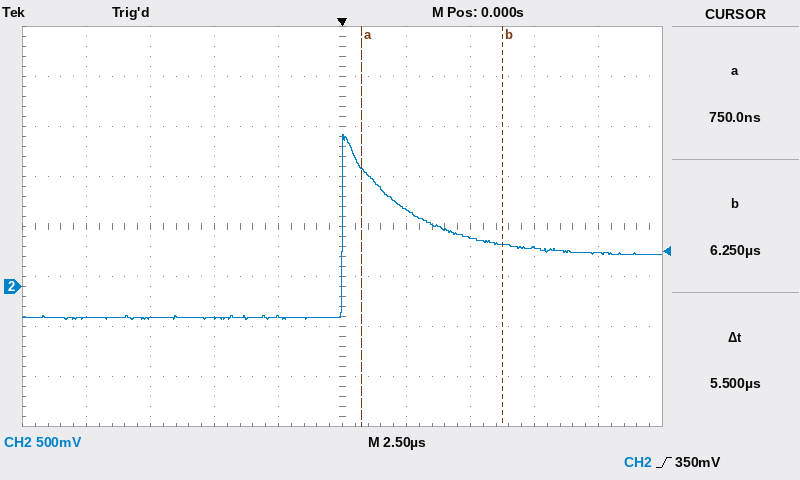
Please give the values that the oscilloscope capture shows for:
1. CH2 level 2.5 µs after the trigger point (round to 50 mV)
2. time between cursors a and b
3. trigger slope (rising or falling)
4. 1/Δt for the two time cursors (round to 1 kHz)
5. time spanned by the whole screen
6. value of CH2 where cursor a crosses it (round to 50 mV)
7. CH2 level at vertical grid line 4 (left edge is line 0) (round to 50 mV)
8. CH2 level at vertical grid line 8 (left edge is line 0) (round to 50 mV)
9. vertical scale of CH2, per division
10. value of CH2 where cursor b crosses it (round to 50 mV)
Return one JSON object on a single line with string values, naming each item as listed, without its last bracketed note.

{"CH2 level 2.5 µs after the trigger point": "750 mV", "time between cursors a and b": "5.5 µs", "trigger slope": "rising", "1/Δt for the two time cursors": "182 kHz", "time spanned by the whole screen": "25 µs", "value of CH2 where cursor a crosses it": "1.20 V", "CH2 level at vertical grid line 4 (left edge is line 0)": "-300 mV", "CH2 level at vertical grid line 8 (left edge is line 0)": "400 mV", "vertical scale of CH2, per division": "500 mV", "value of CH2 where cursor b crosses it": "400 mV"}
